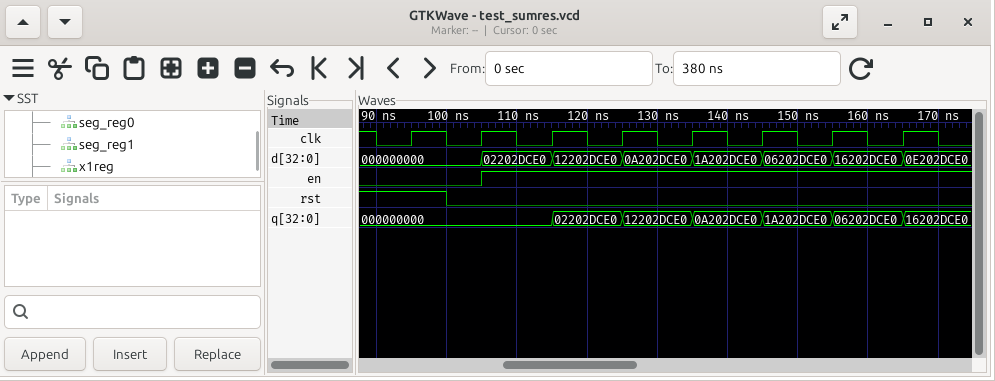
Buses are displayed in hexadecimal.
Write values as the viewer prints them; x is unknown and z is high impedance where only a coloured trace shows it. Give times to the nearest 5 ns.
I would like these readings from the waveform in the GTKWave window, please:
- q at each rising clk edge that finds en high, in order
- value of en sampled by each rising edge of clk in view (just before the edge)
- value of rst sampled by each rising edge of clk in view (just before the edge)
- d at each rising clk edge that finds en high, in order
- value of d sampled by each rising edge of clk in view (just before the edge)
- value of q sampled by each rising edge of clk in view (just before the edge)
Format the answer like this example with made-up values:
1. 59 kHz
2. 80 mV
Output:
1. 000000000, 02202DCE0, 12202DCE0, 0A202DCE0, 1A202DCE0, 06202DCE0
2. 0 0 1 1 1 1 1 1
3. 1 0 0 0 0 0 0 0
4. 02202DCE0, 12202DCE0, 0A202DCE0, 1A202DCE0, 06202DCE0, 16202DCE0
5. 000000000, 000000000, 02202DCE0, 12202DCE0, 0A202DCE0, 1A202DCE0, 06202DCE0, 16202DCE0
6. 000000000, 000000000, 000000000, 02202DCE0, 12202DCE0, 0A202DCE0, 1A202DCE0, 06202DCE0
